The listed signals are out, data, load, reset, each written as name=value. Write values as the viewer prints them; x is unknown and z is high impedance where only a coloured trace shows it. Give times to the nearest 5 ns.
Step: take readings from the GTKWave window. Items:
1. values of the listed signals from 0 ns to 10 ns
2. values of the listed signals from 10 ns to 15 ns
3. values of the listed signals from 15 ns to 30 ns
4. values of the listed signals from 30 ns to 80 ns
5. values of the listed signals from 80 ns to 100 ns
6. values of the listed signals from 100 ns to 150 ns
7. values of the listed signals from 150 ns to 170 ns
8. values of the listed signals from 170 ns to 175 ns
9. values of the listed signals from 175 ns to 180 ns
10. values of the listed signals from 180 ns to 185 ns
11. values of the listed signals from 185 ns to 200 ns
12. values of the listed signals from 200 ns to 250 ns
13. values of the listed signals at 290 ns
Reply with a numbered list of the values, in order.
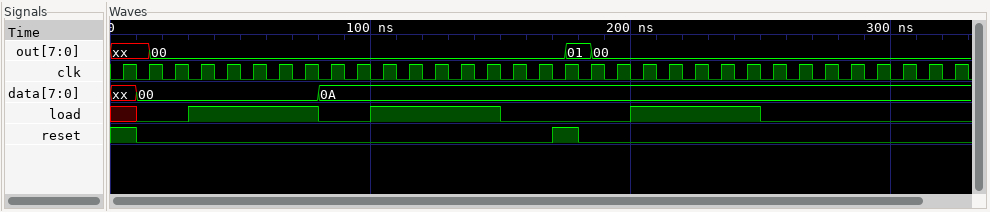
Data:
1. out=xx, data=xx, load=x, reset=1
2. out=xx, data=00, load=0, reset=0
3. out=00, data=00, load=0, reset=0
4. out=00, data=00, load=1, reset=0
5. out=00, data=0A, load=0, reset=0
6. out=00, data=0A, load=1, reset=0
7. out=00, data=0A, load=0, reset=0
8. out=00, data=0A, load=0, reset=1
9. out=01, data=0A, load=0, reset=1
10. out=01, data=0A, load=0, reset=0
11. out=00, data=0A, load=0, reset=0
12. out=00, data=0A, load=1, reset=0
13. out=00, data=0A, load=0, reset=0
